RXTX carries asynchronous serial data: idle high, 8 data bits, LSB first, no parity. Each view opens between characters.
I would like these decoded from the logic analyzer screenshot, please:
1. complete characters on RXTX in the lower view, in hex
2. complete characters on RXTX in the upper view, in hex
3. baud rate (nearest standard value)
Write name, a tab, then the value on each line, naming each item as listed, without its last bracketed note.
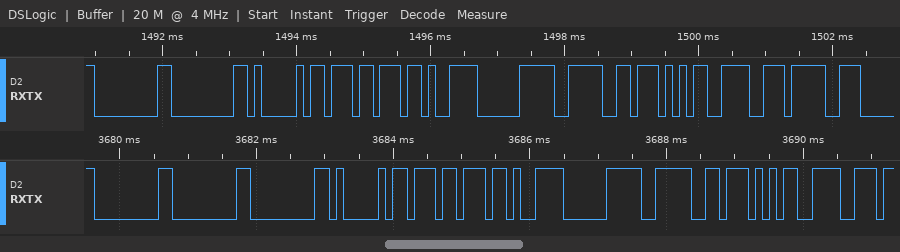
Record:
complete characters on RXTX in the lower view, in hex	00, 00, 00, 41, B7, CB, E0, 3E, 57, 9E
complete characters on RXTX in the upper view, in hex	00, 00, 41, B7, CB, E0, 3E, 57, 9E, 9F
baud rate	9600 baud
